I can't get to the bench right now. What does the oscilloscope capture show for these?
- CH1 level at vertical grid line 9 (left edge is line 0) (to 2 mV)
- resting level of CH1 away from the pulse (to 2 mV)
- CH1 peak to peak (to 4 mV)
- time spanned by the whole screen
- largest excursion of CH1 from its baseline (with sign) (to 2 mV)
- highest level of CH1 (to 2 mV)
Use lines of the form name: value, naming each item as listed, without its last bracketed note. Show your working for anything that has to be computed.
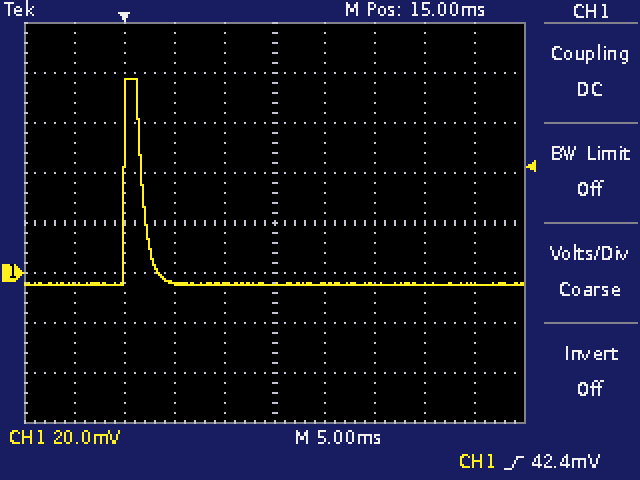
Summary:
CH1 level at vertical grid line 9 (left edge is line 0): -4 mV
resting level of CH1 away from the pulse: -4 mV
CH1 peak to peak: 84 mV
time spanned by the whole screen: 50 ms
largest excursion of CH1 from its baseline (with sign): 78 mV − (-4 mV) = +82 mV
highest level of CH1: 78 mV
